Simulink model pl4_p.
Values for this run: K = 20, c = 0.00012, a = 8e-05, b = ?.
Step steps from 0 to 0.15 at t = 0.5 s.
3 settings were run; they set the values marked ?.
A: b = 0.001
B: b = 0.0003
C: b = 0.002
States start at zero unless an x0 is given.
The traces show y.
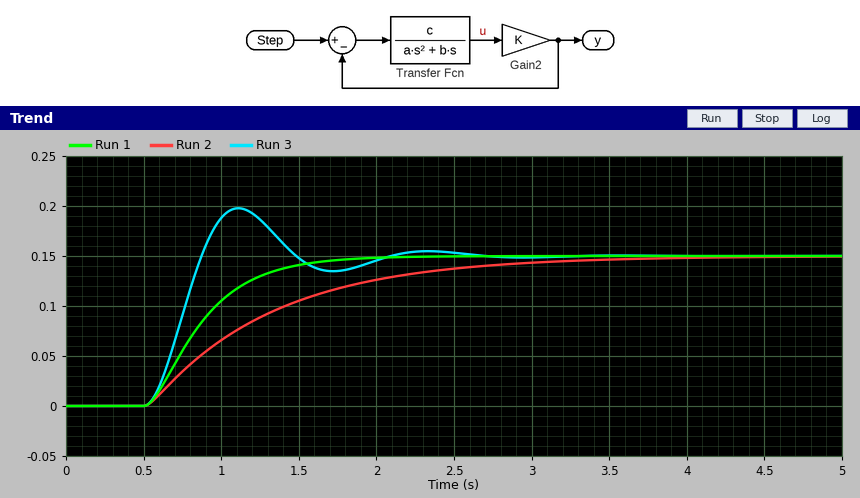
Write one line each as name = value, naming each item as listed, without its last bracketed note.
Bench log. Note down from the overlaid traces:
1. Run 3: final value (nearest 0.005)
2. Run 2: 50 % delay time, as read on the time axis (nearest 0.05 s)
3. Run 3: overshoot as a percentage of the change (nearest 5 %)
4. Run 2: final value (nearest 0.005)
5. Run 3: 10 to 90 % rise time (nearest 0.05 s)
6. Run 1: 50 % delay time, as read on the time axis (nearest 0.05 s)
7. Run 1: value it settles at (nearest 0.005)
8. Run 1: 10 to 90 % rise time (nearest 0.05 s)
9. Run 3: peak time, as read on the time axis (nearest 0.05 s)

Run 3: final value = 0.150
Run 2: 50 % delay time, as read on the time axis = 1.10 s
Run 3: overshoot as a percentage of the change = 30 %
Run 2: final value = 0.150
Run 3: 10 to 90 % rise time = 0.25 s
Run 1: 50 % delay time, as read on the time axis = 0.85 s
Run 1: value it settles at = 0.150
Run 1: 10 to 90 % rise time = 0.75 s
Run 3: peak time, as read on the time axis = 1.10 s
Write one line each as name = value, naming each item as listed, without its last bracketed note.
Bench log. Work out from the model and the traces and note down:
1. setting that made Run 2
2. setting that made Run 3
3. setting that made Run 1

setting that made Run 2 = C
setting that made Run 3 = B
setting that made Run 1 = A
